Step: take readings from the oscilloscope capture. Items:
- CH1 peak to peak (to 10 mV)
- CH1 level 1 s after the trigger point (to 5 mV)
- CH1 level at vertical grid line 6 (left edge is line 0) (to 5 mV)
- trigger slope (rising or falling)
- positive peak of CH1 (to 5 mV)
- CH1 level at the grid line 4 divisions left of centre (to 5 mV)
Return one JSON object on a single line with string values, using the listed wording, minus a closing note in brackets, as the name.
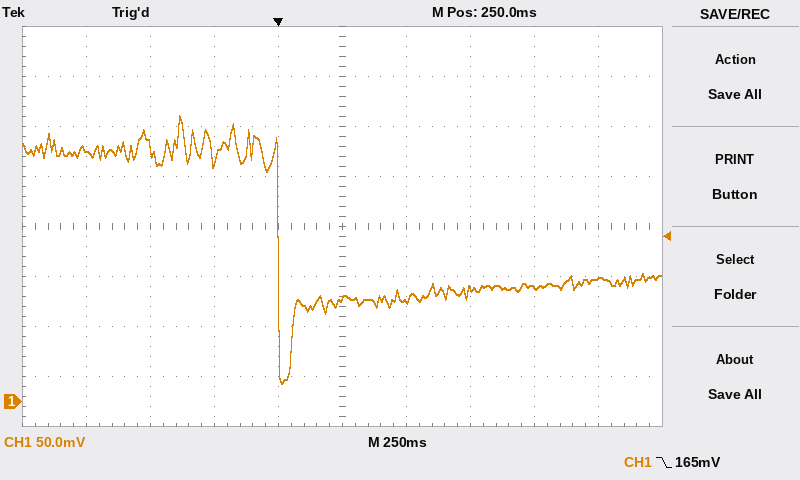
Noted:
{"CH1 peak to peak": "270 mV", "CH1 level 1 s after the trigger point": "115 mV", "CH1 level at vertical grid line 6 (left edge is line 0)": "100 mV", "trigger slope": "falling", "positive peak of CH1": "285 mV", "CH1 level at the grid line 4 divisions left of centre": "250 mV"}
